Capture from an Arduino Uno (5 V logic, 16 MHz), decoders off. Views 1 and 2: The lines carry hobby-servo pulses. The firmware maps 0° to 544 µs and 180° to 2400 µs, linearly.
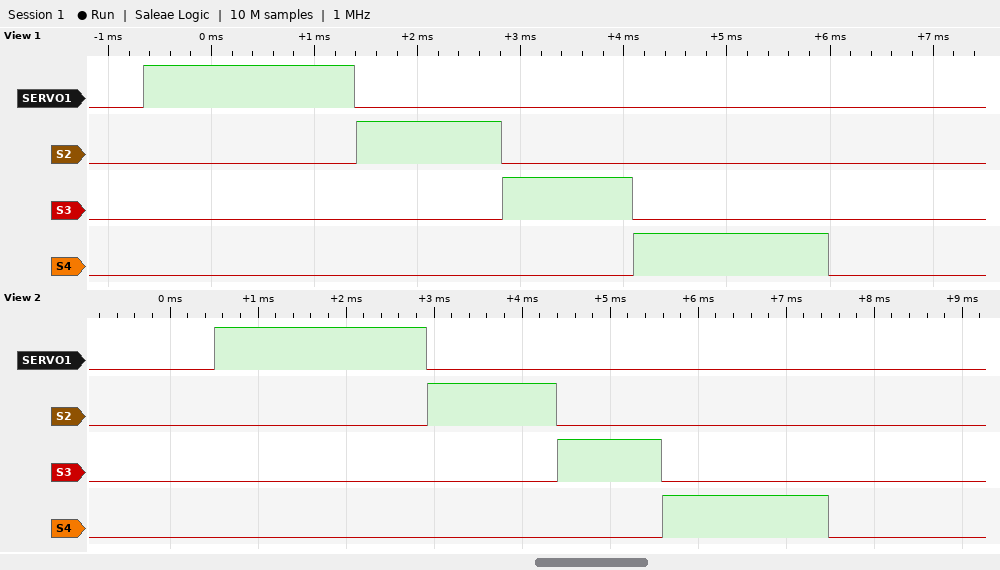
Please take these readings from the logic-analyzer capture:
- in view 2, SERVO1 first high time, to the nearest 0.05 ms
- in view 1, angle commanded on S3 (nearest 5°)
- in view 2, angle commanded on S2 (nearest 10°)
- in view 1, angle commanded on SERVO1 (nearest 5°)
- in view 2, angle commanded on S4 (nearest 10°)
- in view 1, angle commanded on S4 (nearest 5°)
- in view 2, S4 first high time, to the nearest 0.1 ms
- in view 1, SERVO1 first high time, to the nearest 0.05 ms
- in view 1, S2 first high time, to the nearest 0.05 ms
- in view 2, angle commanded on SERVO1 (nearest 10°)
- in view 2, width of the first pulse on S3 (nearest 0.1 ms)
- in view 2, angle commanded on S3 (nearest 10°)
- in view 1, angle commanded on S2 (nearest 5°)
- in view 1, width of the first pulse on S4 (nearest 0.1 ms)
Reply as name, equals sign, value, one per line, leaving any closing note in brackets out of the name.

in view 2, SERVO1 first high time, to the nearest 0.05 ms = 2.40 ms
in view 1, angle commanded on S3 = 70°
in view 2, angle commanded on S2 = 90°
in view 1, angle commanded on SERVO1 = 145°
in view 2, angle commanded on S4 = 130°
in view 1, angle commanded on S4 = 130°
in view 2, S4 first high time, to the nearest 0.1 ms = 1.9 ms
in view 1, SERVO1 first high time, to the nearest 0.05 ms = 2.05 ms
in view 1, S2 first high time, to the nearest 0.05 ms = 1.40 ms
in view 2, angle commanded on SERVO1 = 180°
in view 2, width of the first pulse on S3 = 1.2 ms
in view 2, angle commanded on S3 = 60°
in view 1, angle commanded on S2 = 85°
in view 1, width of the first pulse on S4 = 1.9 ms
